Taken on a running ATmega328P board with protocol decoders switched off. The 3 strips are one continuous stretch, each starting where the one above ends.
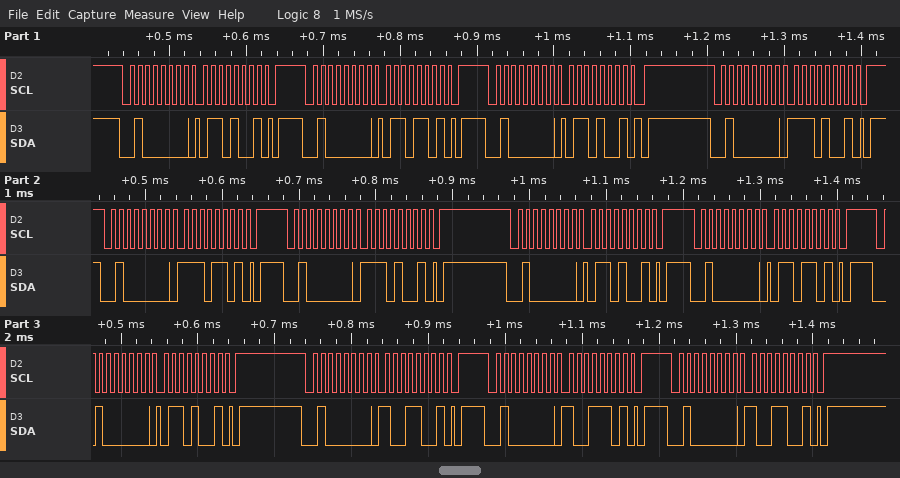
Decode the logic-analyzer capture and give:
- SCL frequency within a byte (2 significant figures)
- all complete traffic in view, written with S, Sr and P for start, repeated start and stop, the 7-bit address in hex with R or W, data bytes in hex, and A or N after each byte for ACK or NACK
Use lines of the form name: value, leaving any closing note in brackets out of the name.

SCL frequency within a byte: 100 kHz
all complete traffic in view, written with S, Sr and P for start, repeated start and stop, the 7-bit address in hex with R or W, data bytes in hex, and A or N after each byte for ACK or NACK: S 20W A 69 A P S 20W A 6D A P S 20W A 69 A P S 20W A E9 A P S 20W A ED A P S 20W A E9 A P S 20W A 69 A P S 20W A 6D A P S 20W A 69 A P S 20W A 99 A P S 20W A 9D A P S 20W A 99 A P
